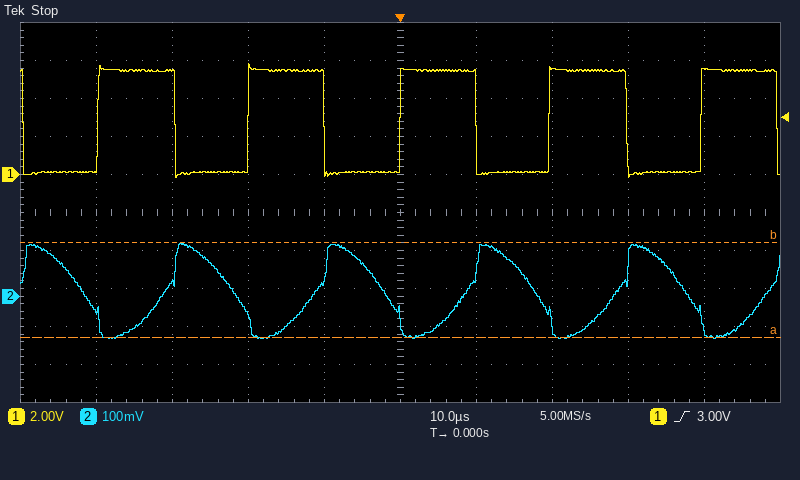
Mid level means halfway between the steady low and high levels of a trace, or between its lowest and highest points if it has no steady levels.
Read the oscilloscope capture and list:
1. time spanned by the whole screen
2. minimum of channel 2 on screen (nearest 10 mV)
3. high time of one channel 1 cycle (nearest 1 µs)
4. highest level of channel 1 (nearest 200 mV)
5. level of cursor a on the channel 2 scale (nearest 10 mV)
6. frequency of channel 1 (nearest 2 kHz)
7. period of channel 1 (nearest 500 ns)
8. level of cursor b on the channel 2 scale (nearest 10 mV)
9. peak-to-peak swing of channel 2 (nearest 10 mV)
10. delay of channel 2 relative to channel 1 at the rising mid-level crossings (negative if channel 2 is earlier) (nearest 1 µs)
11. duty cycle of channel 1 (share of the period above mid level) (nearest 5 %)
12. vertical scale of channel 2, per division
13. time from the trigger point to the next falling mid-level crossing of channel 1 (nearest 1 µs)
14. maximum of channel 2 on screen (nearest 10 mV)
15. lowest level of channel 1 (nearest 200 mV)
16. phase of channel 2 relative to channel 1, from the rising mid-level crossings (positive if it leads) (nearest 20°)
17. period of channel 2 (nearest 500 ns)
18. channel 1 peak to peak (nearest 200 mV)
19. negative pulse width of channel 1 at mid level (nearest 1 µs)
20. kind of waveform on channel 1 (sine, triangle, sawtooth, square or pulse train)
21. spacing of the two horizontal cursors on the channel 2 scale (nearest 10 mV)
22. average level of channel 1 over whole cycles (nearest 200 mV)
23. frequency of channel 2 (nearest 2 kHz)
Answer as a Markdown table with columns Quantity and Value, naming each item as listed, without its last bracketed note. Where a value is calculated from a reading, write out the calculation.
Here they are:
| Quantity | Value |
|---|---|
| time spanned by the whole screen | 100 µs |
| minimum of channel 2 on screen | -110 mV |
| high time of one channel 1 cycle | 10 µs |
| highest level of channel 1 | 5.8 V |
| level of cursor a on the channel 2 scale | -110 mV |
| frequency of channel 1 | 1 / 20.0 µs ≈ 50 kHz |
| period of channel 1 | 20.0 µs |
| level of cursor b on the channel 2 scale | 140 mV |
| peak-to-peak swing of channel 2 | 140 mV − (-110 mV) = 250 mV |
| delay of channel 2 relative to channel 1 at the rising mid-level crossings (negative if channel 2 is earlier) | +9 µs |
| duty cycle of channel 1 (share of the period above mid level) | 10 µs / 20.0 µs ≈ 50 % |
| vertical scale of channel 2, per division | 100 mV |
| time from the trigger point to the next falling mid-level crossing of channel 1 | 10 µs |
| maximum of channel 2 on screen | 140 mV |
| lowest level of channel 1 | -200 mV |
| phase of channel 2 relative to channel 1, from the rising mid-level crossings (positive if it leads) | −360° × (+9 µs) / 20.0 µs ≈ -162°, so -160° to the nearest 20° |
| period of channel 2 | 20.0 µs |
| channel 1 peak to peak | 5.8 V − (-200 mV) = 6.0 V |
| negative pulse width of channel 1 at mid level | 10 µs |
| kind of waveform on channel 1 | square |
| spacing of the two horizontal cursors on the channel 2 scale | 250 mV |
| average level of channel 1 over whole cycles | -200 mV + 0.5 × (5.8 V − (-200 mV)) ≈ 2.8 V |
| frequency of channel 2 | 1 / 20.0 µs ≈ 50 kHz |
